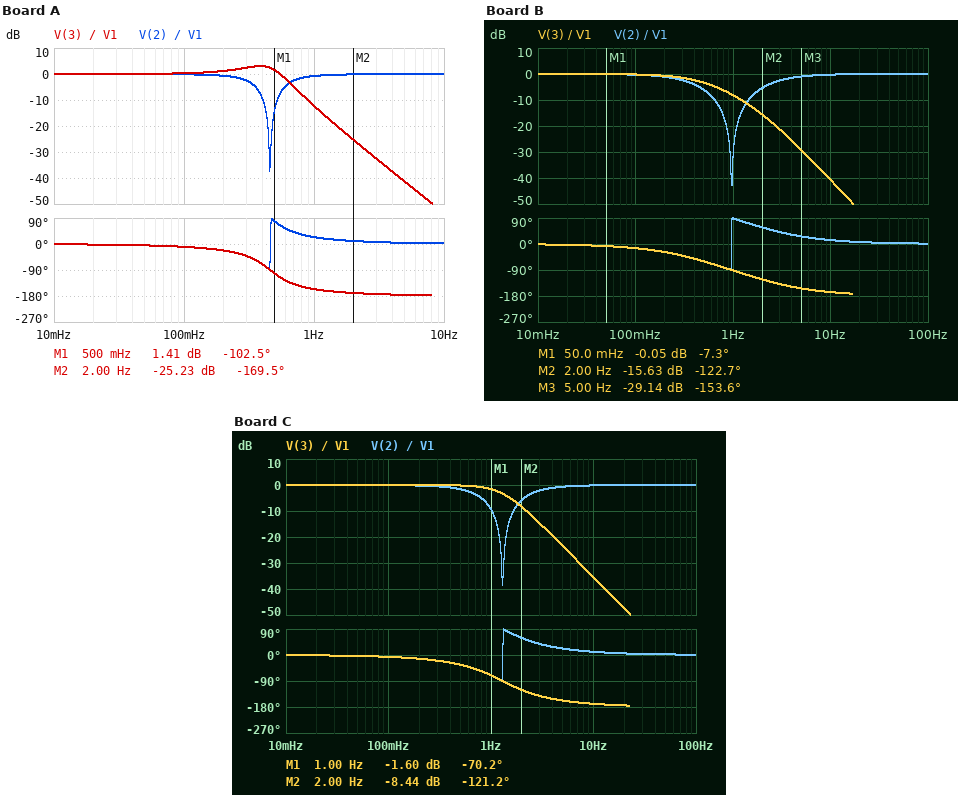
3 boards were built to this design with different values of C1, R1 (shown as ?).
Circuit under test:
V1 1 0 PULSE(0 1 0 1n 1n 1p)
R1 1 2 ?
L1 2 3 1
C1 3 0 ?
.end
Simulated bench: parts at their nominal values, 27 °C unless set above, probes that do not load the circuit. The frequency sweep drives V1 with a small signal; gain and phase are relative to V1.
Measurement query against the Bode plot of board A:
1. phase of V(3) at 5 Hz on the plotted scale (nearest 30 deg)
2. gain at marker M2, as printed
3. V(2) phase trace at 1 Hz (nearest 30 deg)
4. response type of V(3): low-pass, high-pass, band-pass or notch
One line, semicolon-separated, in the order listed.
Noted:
-180 deg; -25.23 dB; 30 deg; low-pass
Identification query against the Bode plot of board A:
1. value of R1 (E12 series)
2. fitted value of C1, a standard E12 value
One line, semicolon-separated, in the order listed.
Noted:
2.2 Ω; 120 mF
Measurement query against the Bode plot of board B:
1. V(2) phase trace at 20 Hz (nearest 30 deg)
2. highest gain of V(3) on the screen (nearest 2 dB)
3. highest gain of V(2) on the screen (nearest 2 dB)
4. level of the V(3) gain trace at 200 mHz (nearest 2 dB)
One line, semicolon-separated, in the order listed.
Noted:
0 deg; 0 dB; 0 dB; 0 dB
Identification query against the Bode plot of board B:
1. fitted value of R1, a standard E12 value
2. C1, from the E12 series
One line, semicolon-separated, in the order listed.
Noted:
15 Ω; 27 mF
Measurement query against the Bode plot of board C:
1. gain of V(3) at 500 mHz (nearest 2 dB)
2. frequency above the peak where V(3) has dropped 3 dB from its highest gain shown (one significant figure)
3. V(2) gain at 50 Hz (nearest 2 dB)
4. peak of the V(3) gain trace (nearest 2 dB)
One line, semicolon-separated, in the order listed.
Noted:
0 dB; 1 Hz; 0 dB; 0 dB
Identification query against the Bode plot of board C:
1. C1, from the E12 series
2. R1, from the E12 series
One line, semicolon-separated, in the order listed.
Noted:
15 mF; 12 Ω
